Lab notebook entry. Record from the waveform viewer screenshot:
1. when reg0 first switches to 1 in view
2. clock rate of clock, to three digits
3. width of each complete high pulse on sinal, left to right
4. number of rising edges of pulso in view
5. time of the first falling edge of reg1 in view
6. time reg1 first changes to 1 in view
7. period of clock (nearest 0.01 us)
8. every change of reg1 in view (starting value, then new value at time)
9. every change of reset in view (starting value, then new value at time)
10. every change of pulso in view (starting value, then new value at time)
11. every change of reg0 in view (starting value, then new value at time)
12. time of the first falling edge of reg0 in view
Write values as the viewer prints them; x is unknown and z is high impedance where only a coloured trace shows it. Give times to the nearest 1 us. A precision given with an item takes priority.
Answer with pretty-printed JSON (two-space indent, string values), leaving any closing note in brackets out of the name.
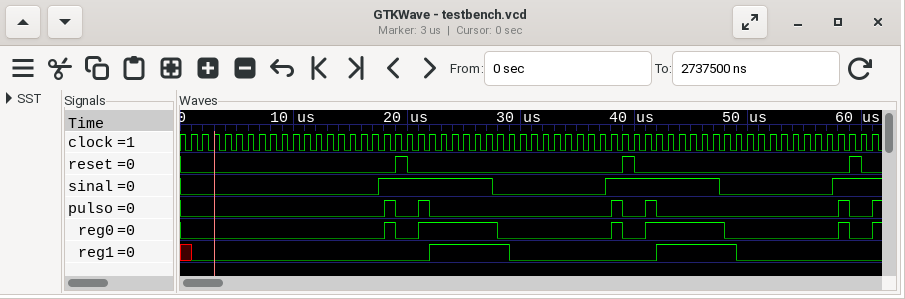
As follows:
{
  "when reg0 first switches to 1 in view": "18 us",
  "clock rate of clock, to three digits": "1.00 MHz",
  "width of each complete high pulse on sinal, left to right": "10 us, 10 us",
  "number of rising edges of pulso in view": "6",
  "time of the first falling edge of reg1 in view": "29 us",
  "time reg1 first changes to 1 in view": "22 us",
  "period of clock": "1 us",
  "every change of reg1 in view": "x, 0 at 1 us, 1 at 22 us, 0 at 29 us, 1 at 42 us, 0 at 49 us",
  "every change of reset in view": "0, 1 at 19 us, 0 at 20 us, 1 at 39 us, 0 at 40 us, 1 at 59 us, 0 at 60 us",
  "every change of pulso in view": "0, 1 at 18 us, 0 at 19 us, 1 at 21 us, 0 at 22 us, 1 at 38 us, 0 at 39 us, 1 at 41 us, 0 at 42 us, 1 at 58 us, 0 at 59 us, 1 at 61 us",
  "every change of reg0 in view": "0, 1 at 18 us, 0 at 19 us, 1 at 21 us, 0 at 28 us, 1 at 38 us, 0 at 39 us, 1 at 41 us, 0 at 48 us, 1 at 58 us, 0 at 59 us, 1 at 61 us",
  "time of the first falling edge of reg0 in view": "19 us"
}
